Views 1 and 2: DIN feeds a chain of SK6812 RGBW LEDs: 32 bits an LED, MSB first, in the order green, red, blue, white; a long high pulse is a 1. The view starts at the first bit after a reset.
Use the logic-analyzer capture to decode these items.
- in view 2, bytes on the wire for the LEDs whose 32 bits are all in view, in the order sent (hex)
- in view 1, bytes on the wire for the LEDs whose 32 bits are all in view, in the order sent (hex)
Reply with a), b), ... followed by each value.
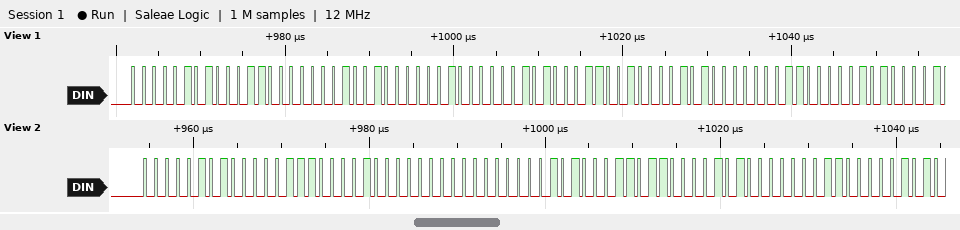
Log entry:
a) 05 07 08 00 05 1B 0A 03
b) 05 18 09 02 05 19 0A 03
